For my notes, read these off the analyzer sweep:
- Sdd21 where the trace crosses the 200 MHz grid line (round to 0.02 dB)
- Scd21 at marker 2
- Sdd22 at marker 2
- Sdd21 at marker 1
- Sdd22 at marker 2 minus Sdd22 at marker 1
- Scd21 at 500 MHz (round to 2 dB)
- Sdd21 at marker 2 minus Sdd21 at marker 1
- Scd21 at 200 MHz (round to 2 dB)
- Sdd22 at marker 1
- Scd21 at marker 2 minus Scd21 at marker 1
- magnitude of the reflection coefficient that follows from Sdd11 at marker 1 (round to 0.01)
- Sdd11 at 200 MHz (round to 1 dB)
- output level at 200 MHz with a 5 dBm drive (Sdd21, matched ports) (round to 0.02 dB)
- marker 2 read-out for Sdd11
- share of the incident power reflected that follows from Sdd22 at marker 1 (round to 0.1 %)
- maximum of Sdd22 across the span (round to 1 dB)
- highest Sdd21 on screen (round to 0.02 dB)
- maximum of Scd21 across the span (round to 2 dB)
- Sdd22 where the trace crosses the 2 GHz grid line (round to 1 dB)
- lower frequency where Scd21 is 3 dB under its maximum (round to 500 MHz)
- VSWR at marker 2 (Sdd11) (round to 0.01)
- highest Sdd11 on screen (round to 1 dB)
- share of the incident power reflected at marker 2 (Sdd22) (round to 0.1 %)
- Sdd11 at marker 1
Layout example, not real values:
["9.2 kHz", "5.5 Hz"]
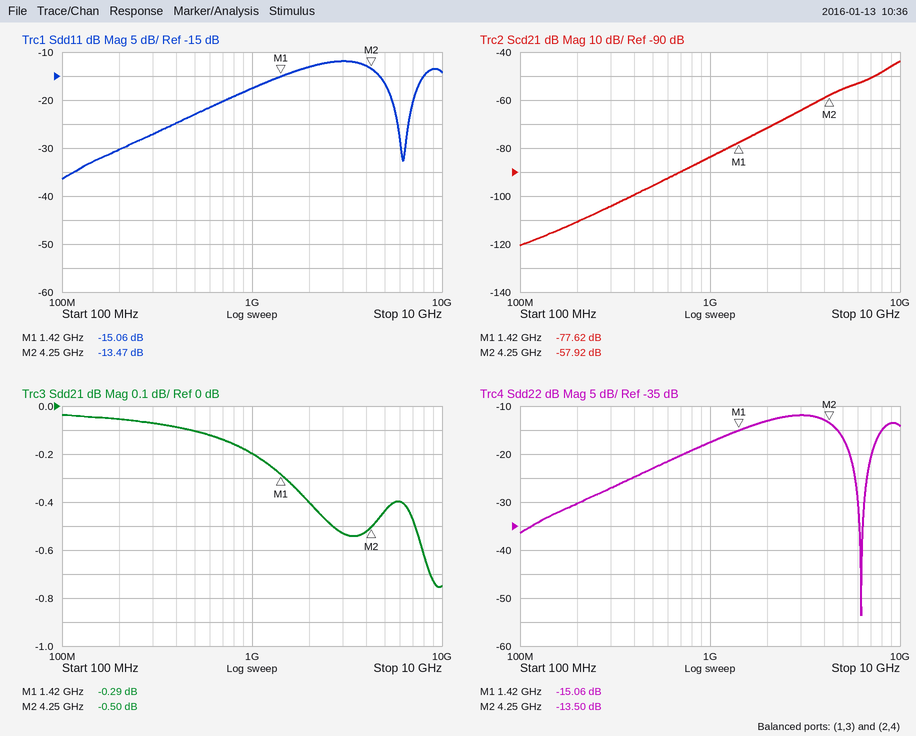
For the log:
["-0.06 dB", "-57.92 dB", "-13.50 dB", "-0.29 dB", "1.56 dB", "-96 dB", "-0.21 dB", "-110 dB", "-15.06 dB", "19.70 dB", "0.18", "-30 dB", "4.94 dBm", "-13.47 dB", "3.1 %", "-12 dB", "-0.04 dB", "-44 dB", "-13 dB", "8.5 GHz", "1.54", "-12 dB", "4.5 %", "-15.06 dB"]
